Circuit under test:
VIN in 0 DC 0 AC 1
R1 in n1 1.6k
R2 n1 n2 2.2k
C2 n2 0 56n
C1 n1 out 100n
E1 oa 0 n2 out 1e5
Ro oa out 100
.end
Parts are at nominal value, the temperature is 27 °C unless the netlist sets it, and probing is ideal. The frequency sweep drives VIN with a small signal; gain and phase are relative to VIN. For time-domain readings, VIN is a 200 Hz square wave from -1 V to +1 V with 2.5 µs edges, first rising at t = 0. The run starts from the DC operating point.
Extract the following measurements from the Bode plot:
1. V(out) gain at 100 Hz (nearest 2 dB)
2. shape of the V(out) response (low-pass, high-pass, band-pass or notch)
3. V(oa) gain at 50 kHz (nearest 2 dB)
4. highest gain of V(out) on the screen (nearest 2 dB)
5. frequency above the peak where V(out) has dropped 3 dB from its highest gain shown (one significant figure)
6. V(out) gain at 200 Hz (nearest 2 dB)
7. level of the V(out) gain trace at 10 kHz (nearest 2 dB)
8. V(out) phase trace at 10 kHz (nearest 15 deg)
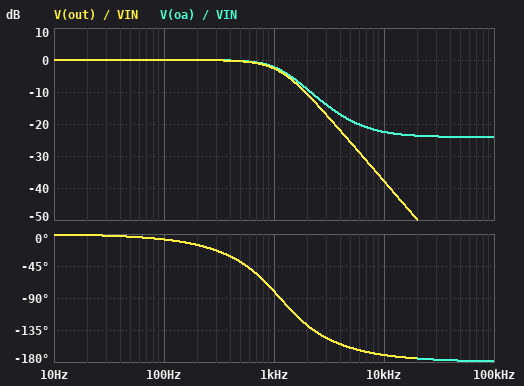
0 dB
low-pass
-24 dB
0 dB
1 kHz
0 dB
-38 dB
-165 deg
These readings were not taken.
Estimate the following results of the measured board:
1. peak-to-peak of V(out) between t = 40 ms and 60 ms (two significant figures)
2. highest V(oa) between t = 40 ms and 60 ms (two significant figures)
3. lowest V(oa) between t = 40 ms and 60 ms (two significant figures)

2.1 V
1.1 V
-1.1 V
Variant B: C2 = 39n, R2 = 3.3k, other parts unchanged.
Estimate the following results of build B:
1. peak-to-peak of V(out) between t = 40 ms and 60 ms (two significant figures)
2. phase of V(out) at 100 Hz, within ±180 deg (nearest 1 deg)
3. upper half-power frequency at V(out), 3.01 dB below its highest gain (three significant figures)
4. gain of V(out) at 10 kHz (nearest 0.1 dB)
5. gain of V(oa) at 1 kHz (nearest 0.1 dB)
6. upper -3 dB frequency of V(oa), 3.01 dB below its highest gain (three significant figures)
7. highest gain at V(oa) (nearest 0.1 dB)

2.2 V
-7 deg
1.17 kHz
-38.2 dB
-1.3 dB
1.23 kHz
0.1 dB
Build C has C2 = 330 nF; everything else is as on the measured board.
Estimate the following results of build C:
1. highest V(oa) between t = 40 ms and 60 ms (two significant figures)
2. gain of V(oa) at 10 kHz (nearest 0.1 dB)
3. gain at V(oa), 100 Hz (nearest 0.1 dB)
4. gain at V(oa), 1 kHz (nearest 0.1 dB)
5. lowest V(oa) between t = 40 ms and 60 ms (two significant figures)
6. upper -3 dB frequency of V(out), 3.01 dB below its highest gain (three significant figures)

900 mV
-23.9 dB
-1.8 dB
-16.6 dB
-900 mV
137 Hz
